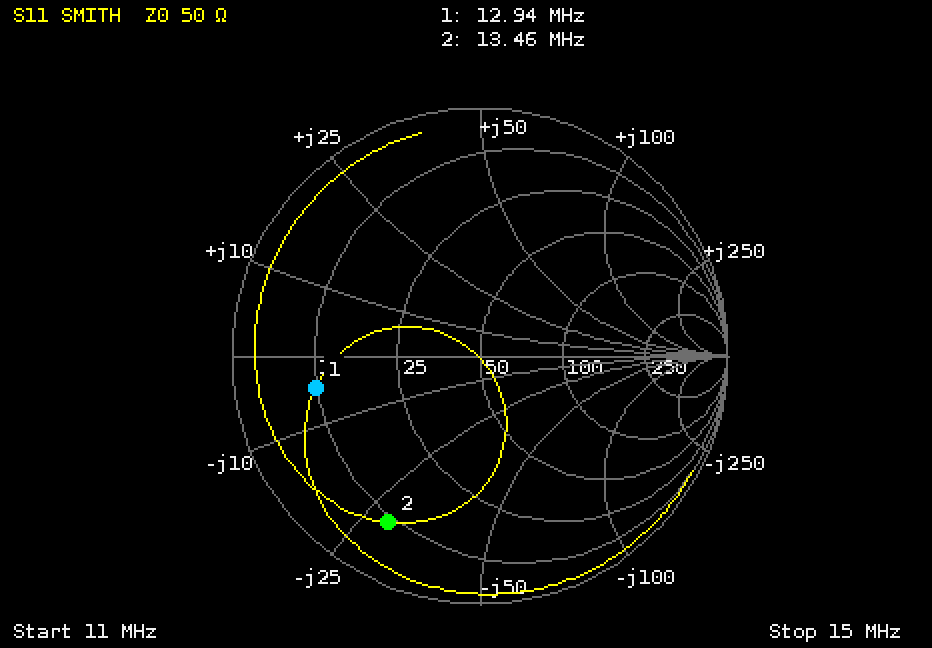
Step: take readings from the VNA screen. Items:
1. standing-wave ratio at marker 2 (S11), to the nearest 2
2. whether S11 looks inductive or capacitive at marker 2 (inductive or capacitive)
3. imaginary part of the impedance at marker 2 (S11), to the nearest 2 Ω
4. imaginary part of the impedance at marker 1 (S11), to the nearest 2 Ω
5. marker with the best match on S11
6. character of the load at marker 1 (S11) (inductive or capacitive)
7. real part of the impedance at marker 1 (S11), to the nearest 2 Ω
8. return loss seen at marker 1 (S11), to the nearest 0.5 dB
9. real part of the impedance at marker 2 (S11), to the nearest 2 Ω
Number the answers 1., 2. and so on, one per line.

1. 8
2. capacitive
3. -28 Ω
4. -4 Ω
5. marker 1
6. capacitive
7. 10 Ω
8. 3.5 dB
9. 8 Ω
